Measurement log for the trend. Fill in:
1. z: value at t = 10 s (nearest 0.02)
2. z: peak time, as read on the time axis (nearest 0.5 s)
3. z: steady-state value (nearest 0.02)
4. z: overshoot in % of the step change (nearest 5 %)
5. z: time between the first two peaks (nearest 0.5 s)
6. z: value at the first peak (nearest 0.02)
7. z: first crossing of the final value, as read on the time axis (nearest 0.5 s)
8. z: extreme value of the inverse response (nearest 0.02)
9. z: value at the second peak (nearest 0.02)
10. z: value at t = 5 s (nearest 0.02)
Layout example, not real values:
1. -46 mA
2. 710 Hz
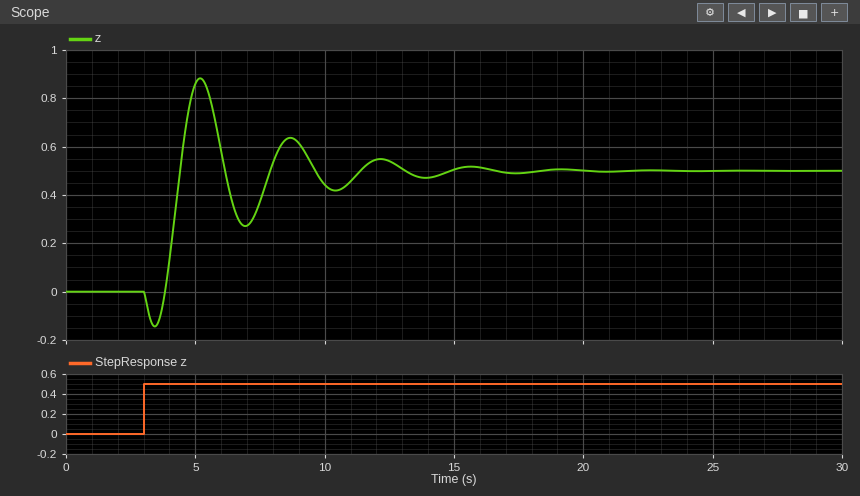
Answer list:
1. 0.44
2. 5.0 s
3. 0.50
4. 75 %
5. 3.5 s
6. 0.88
7. 4.5 s
8. -0.14
9. 0.64
10. 0.86
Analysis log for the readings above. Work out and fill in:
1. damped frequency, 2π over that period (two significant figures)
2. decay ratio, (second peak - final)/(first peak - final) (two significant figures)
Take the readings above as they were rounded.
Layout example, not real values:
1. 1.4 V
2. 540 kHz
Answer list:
1. 1.8 rad/s
2. 0.37
